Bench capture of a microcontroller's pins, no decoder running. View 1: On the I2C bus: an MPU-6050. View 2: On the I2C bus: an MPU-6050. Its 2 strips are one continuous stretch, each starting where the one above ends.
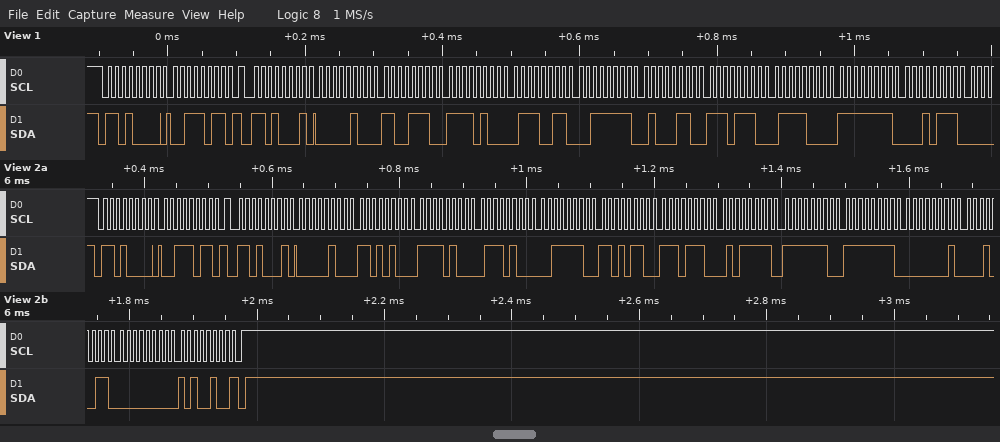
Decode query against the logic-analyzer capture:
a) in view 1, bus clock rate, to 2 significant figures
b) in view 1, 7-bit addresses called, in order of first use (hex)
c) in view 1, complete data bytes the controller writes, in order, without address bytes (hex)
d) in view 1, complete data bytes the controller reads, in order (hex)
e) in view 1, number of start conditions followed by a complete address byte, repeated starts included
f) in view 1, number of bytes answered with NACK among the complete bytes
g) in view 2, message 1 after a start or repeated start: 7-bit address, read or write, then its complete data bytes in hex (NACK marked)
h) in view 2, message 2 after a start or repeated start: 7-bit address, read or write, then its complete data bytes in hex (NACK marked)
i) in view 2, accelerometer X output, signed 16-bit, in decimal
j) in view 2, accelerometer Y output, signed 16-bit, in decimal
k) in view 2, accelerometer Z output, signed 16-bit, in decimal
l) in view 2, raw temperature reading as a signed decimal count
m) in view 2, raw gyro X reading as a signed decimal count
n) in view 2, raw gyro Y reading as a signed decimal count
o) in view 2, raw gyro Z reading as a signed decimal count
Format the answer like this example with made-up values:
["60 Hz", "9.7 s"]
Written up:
["100 kHz", "0x68", "3B", "04 CE F4 73 3F 46 EE 78 FF 17", "2", "0", "0x68 write: 3B", "0x68 read: 04 D4 F4 74 3E D6 EE 5F FE FF 01 13 00 A4 NACK", "1236", "-2956", "16086", "-4513", "-257", "275", "164"]
